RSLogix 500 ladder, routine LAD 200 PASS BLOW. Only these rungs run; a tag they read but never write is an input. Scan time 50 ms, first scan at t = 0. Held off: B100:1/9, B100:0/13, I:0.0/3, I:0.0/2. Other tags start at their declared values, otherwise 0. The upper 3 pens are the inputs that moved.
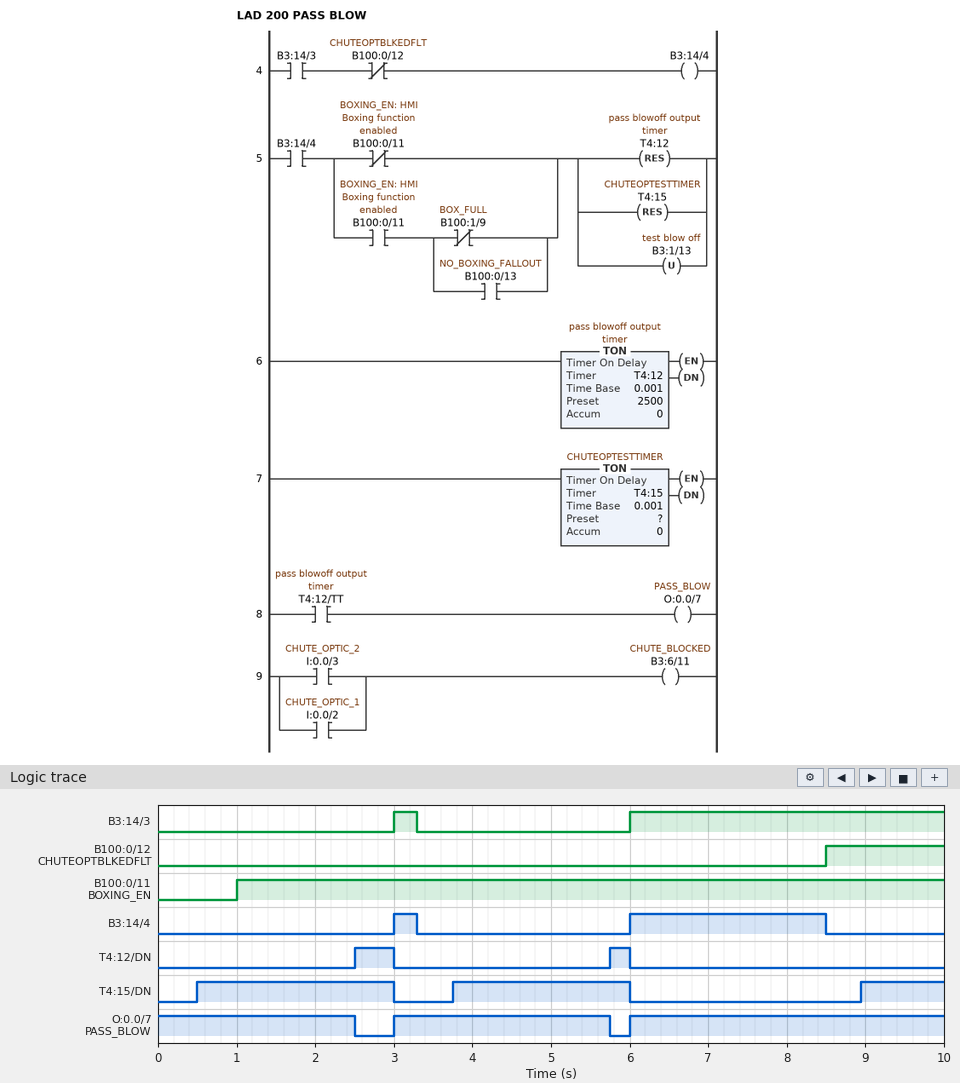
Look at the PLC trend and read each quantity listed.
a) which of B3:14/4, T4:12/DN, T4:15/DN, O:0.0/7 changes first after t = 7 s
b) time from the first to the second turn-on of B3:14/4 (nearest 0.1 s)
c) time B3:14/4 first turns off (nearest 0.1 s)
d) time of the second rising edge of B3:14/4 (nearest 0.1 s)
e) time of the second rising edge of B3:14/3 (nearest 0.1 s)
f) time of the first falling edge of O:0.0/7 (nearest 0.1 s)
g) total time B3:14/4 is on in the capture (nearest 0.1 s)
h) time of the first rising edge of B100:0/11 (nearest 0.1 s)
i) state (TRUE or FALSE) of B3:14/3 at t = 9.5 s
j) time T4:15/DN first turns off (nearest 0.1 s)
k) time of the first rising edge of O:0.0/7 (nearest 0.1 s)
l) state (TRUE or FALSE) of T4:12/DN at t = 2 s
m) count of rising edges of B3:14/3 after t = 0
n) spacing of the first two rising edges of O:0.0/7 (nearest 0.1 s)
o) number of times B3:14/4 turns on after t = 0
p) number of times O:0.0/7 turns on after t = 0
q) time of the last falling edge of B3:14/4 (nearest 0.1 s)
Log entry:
B3:14/4
3.0 s
3.3 s
6.0 s
6.0 s
2.5 s
2.8 s
1.0 s
TRUE
3.0 s
3.0 s
FALSE
2
3.0 s
2
2
8.5 s
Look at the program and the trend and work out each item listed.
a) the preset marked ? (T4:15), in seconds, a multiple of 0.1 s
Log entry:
0.5 s
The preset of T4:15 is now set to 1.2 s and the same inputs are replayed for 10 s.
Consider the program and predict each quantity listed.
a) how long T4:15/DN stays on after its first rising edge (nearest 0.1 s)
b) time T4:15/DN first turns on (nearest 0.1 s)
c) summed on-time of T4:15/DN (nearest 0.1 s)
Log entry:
1.8 s
1.2 s
3.7 s
